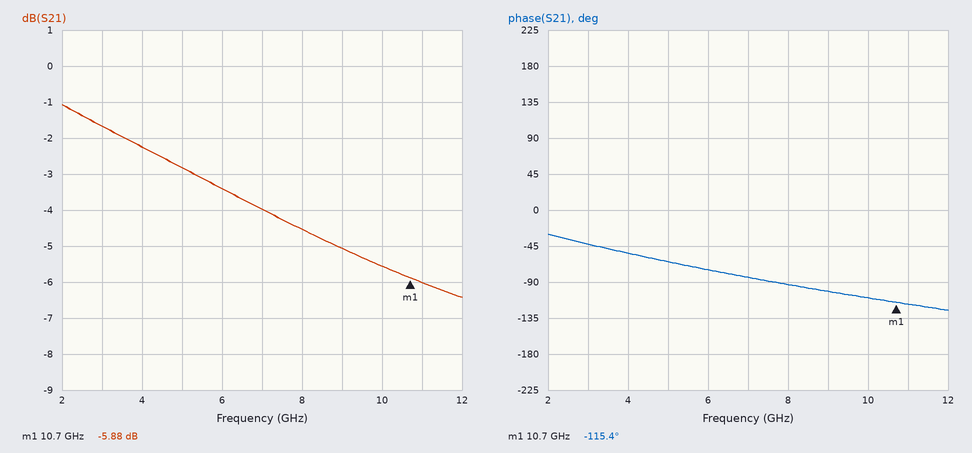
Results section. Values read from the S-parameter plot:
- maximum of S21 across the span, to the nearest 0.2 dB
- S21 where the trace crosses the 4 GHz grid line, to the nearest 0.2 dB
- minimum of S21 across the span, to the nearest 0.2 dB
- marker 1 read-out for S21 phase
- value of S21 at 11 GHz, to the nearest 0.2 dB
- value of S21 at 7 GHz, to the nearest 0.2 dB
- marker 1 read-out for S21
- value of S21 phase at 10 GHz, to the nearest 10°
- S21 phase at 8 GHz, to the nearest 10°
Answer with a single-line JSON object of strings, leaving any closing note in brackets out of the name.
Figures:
{"maximum of S21 across the span, to the nearest 0.2 dB": "-1.0 dB", "S21 where the trace crosses the 4 GHz grid line, to the nearest 0.2 dB": "-2.2 dB", "minimum of S21 across the span, to the nearest 0.2 dB": "-6.4 dB", "marker 1 read-out for S21 phase": "-115.4°", "value of S21 at 11 GHz, to the nearest 0.2 dB": "-6.0 dB", "value of S21 at 7 GHz, to the nearest 0.2 dB": "-4.0 dB", "marker 1 read-out for S21": "-5.88 dB", "value of S21 phase at 10 GHz, to the nearest 10°": "-110°", "S21 phase at 8 GHz, to the nearest 10°": "-90°"}
